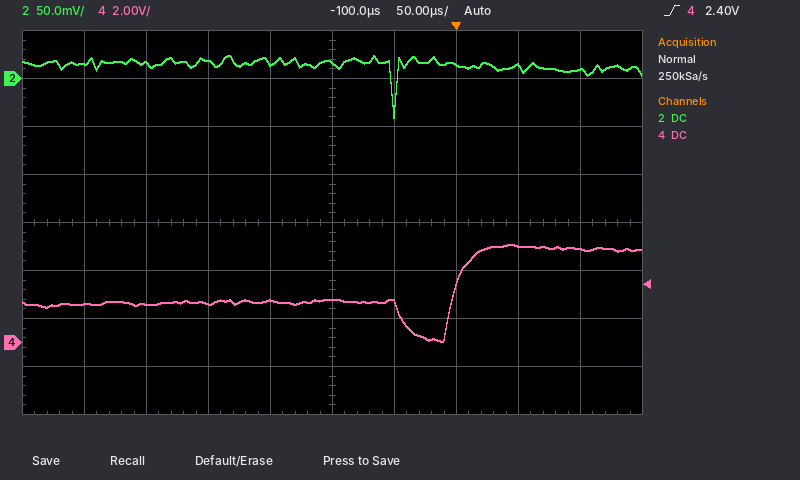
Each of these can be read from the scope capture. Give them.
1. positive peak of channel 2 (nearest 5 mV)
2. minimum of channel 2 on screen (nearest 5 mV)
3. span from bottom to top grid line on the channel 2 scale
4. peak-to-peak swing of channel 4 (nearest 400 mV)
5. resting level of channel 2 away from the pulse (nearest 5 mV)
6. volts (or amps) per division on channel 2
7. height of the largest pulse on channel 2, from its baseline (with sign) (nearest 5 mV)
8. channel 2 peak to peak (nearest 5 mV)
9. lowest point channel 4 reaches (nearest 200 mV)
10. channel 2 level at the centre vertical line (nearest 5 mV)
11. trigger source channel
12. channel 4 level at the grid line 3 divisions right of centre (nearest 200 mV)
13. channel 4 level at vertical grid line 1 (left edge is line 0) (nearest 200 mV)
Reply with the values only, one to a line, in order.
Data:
25 mV
-40 mV
400 mV
4.0 V
15 mV
50 mV
-55 mV
65 mV
0.0 V
15 mV
channel 4
4.0 V
1.6 V
